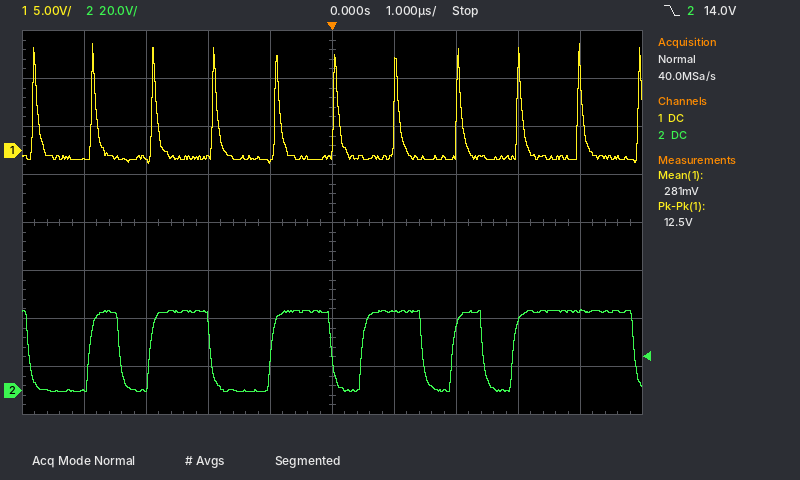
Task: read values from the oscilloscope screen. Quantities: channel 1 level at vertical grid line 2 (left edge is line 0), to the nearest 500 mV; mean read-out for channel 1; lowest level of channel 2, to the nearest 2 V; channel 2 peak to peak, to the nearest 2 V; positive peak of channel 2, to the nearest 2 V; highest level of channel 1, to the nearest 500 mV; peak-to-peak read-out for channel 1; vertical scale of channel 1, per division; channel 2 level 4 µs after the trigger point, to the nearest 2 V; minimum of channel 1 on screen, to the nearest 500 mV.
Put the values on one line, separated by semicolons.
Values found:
-1.0 V; 281 mV; 0 V; 34 V; 34 V; 11.0 V; 12.5 V; 5 V; 34 V; -1.5 V
